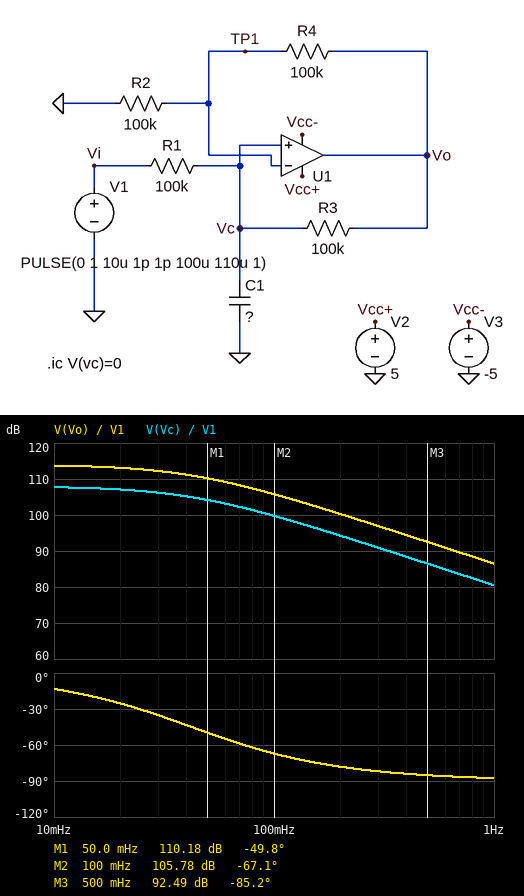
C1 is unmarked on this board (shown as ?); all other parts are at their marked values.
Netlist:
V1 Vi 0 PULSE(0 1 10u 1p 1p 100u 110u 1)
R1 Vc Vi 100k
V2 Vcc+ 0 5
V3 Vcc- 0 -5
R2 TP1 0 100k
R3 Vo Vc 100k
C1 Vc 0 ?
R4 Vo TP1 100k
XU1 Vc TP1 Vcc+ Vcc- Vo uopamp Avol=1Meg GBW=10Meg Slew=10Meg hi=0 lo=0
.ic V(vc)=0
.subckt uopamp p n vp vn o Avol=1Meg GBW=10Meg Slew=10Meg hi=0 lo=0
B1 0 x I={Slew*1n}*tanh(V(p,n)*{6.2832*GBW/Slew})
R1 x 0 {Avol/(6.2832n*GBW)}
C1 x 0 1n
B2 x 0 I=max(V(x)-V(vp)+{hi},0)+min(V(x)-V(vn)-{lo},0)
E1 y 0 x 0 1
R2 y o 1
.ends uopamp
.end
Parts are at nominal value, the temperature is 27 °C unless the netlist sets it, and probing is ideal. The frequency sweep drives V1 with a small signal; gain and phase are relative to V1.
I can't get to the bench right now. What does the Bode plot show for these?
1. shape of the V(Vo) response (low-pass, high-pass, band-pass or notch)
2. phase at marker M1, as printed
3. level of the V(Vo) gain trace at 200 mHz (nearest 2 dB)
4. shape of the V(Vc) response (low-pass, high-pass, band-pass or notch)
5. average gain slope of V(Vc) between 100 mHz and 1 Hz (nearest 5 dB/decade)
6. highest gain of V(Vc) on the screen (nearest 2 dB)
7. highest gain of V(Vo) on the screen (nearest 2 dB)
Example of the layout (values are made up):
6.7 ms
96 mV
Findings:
low-pass
-49.8 deg
100 dB
low-pass
-20 dB/decade
108 dB
114 dB
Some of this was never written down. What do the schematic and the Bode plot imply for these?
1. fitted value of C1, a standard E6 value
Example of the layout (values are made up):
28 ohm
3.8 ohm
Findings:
150 pF
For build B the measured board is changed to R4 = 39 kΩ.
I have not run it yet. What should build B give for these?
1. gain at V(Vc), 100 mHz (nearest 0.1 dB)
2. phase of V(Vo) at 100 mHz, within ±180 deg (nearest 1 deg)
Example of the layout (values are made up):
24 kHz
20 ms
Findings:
4.3 dB
0 deg
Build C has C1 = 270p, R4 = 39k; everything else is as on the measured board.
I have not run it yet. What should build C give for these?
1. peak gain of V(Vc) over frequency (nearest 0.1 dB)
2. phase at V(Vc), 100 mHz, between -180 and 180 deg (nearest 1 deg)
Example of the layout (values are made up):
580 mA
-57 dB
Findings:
4.3 dB
0 deg
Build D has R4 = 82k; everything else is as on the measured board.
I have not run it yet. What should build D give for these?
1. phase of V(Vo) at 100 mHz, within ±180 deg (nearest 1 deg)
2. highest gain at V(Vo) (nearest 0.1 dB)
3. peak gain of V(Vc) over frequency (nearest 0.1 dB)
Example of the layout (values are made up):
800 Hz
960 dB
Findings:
0 deg
20.1 dB
14.9 dB
